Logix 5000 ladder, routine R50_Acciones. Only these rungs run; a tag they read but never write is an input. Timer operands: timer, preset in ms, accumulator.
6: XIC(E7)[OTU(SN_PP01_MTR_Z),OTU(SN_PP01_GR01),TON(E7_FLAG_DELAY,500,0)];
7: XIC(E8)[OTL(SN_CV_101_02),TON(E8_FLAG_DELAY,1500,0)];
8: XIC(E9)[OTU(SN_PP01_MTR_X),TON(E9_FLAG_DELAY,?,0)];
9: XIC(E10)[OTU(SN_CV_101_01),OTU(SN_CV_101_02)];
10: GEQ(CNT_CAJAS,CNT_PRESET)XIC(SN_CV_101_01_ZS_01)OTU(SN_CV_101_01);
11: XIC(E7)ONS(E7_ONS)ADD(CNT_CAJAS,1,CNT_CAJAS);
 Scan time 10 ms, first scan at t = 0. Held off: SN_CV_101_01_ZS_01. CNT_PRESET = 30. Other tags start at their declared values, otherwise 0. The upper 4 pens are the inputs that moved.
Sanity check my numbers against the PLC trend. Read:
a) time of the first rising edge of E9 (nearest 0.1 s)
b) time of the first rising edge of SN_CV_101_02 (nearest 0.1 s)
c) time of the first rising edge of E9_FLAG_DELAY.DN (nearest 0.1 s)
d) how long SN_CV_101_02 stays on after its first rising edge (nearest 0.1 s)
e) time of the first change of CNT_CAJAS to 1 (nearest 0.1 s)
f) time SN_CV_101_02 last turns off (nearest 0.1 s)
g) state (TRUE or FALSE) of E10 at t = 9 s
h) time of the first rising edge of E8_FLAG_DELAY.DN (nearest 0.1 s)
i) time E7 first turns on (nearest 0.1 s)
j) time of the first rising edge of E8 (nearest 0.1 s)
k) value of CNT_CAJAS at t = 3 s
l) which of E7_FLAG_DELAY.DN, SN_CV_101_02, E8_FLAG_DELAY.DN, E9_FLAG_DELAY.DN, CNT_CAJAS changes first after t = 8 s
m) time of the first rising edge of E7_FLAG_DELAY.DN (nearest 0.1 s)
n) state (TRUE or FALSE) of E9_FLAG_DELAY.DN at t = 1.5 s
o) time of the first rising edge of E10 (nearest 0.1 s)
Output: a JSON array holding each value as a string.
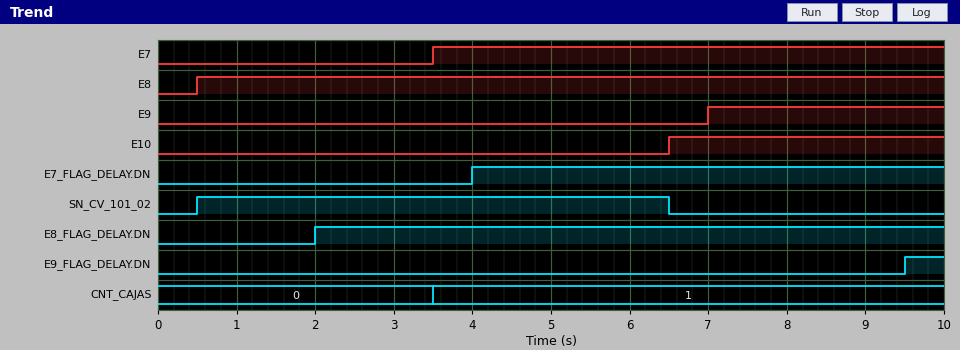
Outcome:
["7.0 s", "0.5 s", "9.5 s", "6.0 s", "3.5 s", "6.5 s", "TRUE", "2.0 s", "3.5 s", "0.5 s", "0", "E9_FLAG_DELAY.DN", "4.0 s", "FALSE", "6.5 s"]
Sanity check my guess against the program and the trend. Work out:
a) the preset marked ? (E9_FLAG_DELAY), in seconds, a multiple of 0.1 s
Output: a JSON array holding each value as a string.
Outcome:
["2.5 s"]
